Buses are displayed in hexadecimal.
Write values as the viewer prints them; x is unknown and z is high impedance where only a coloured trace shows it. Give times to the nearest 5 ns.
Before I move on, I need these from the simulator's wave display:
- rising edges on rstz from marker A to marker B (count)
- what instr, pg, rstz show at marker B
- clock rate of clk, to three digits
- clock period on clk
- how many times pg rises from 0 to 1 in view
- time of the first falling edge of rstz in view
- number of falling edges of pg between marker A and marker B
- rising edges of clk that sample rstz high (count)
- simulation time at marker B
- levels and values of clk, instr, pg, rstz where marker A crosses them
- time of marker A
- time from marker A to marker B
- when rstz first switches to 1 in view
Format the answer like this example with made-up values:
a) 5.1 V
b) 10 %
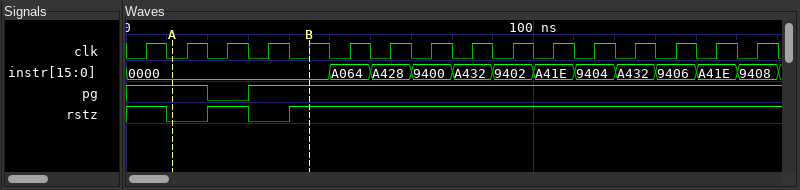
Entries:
a) 2
b) instr=0000, pg=1, rstz=1
c) 100 MHz
d) 10 ns
e) 1
f) 10 ns
g) 1
h) 14
i) 45 ns
j) clk=0, instr=0000, pg=1, rstz=0
k) 10 ns
l) 35 ns
m) 20 ns
